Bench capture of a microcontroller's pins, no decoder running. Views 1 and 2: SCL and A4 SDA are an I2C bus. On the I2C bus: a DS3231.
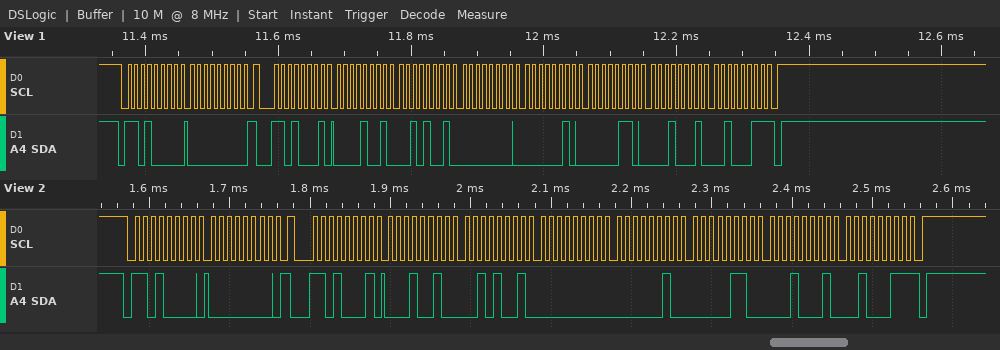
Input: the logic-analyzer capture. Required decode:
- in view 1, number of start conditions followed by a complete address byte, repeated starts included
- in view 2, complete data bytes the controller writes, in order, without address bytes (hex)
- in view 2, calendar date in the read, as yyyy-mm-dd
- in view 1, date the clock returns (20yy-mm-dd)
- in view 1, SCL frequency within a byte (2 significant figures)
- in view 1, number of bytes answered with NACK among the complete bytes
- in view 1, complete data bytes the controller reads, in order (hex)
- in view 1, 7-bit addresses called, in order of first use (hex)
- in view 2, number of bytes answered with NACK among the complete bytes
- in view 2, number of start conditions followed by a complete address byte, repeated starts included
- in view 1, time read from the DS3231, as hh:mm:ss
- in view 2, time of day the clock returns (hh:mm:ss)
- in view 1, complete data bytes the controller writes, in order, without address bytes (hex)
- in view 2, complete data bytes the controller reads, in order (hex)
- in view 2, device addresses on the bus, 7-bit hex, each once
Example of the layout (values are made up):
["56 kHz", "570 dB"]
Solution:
["2", "00", "2023-11-06", "2023-11-06", "100 kHz", "1", "09 29 00 02 06 11 23", "0x68", "1", "2", "00:29:09", "00:29:12", "00", "12 29 00 02 06 11 23", "0x68"]
